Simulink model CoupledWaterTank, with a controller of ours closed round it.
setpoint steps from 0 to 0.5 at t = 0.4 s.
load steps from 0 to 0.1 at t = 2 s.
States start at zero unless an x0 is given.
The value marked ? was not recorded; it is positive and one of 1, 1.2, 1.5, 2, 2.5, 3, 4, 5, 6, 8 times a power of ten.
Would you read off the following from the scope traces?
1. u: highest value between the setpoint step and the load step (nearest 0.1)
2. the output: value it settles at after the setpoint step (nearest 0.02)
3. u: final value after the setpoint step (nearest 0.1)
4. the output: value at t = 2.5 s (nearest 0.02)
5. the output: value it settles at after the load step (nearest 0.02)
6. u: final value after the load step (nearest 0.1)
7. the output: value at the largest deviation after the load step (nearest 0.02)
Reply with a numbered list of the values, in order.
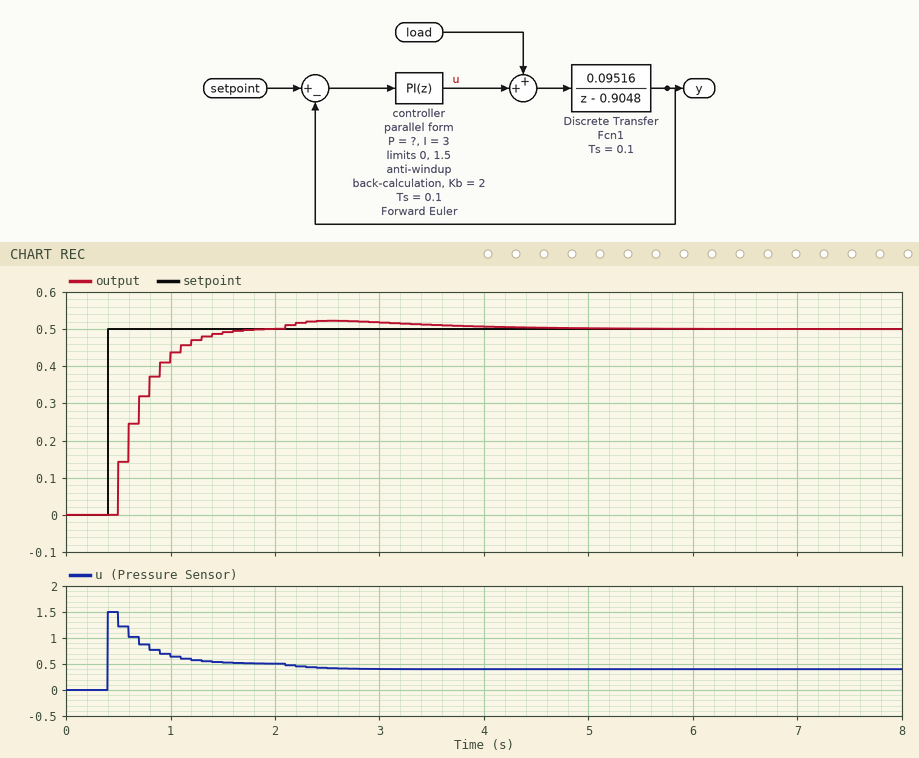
1. 1.5
2. 0.50
3. 0.5
4. 0.52
5. 0.50
6. 0.4
7. 0.52
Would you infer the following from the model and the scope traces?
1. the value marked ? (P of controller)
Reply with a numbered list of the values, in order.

1. 3
